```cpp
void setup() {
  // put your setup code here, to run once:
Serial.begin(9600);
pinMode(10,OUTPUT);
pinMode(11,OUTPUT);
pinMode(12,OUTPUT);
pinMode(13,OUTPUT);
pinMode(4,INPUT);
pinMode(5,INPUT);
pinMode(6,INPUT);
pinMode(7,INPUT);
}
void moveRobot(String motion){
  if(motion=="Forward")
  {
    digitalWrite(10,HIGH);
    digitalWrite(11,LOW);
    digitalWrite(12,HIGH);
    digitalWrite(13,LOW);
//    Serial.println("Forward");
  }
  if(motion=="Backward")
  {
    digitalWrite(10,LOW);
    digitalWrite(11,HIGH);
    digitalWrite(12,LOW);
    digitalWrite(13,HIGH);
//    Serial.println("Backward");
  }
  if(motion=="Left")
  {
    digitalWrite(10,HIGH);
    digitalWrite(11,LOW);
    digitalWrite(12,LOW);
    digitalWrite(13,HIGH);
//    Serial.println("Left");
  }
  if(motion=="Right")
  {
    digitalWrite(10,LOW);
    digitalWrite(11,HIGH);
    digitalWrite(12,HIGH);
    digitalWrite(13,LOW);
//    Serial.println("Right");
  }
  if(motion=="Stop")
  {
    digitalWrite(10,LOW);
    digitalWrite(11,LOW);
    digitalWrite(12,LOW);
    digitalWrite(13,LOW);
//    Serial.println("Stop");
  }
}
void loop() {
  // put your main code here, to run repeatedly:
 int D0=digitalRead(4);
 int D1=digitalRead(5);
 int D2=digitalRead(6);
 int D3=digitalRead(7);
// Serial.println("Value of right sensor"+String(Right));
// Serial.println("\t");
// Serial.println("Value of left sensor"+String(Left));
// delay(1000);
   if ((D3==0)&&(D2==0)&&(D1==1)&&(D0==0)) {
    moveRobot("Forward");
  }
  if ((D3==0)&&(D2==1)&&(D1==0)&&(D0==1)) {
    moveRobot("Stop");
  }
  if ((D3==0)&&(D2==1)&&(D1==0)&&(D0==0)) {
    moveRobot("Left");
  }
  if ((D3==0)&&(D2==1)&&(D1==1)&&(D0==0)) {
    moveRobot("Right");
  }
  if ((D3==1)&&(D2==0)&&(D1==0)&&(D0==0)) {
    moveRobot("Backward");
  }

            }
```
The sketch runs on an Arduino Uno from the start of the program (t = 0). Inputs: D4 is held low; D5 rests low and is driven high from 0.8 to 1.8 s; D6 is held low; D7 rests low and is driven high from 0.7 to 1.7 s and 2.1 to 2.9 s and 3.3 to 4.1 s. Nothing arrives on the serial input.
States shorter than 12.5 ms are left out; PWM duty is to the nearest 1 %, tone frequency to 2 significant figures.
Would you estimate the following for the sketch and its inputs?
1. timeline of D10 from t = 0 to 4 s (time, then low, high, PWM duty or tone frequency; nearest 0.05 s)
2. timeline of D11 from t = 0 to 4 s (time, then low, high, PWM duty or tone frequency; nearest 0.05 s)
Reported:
0 s low; 1.7 s high; 2.1 s low
0 s low; 0.7 s high; 1.7 s low; 2.1 s high
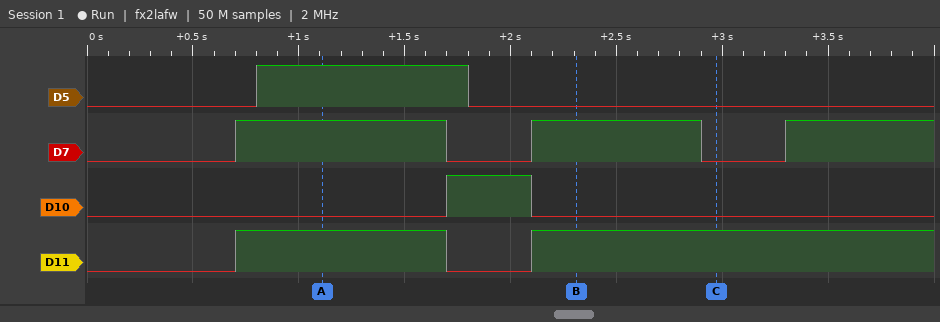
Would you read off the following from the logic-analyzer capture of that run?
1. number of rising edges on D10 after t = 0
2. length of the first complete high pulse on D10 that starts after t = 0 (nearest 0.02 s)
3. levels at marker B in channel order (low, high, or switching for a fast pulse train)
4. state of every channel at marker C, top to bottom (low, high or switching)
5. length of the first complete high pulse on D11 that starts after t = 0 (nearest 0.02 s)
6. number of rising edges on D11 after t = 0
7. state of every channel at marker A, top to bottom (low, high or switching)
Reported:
1
0.40 s
D5 low, D7 high, D10 low, D11 high
D5 low, D7 low, D10 low, D11 high
1.00 s
2
D5 high, D7 high, D10 low, D11 high
